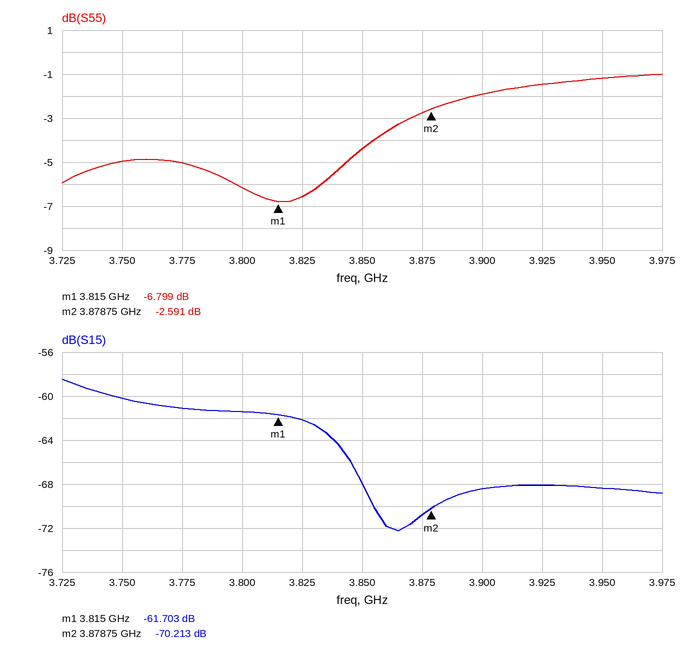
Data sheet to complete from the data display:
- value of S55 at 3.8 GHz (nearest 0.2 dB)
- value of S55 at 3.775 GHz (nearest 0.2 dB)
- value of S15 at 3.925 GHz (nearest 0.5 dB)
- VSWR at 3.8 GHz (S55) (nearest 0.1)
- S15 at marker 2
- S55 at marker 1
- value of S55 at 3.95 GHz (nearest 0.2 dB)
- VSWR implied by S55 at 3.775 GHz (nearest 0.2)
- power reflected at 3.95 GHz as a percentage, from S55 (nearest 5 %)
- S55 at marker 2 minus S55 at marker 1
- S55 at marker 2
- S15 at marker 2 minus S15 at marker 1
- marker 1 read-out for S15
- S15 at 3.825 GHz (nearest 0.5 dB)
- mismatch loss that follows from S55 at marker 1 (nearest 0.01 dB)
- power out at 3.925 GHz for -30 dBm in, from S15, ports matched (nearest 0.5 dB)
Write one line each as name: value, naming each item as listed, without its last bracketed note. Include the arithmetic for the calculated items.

value of S55 at 3.8 GHz: -6.2 dB
value of S55 at 3.775 GHz: -5.0 dB
value of S15 at 3.925 GHz: -68.0 dB
VSWR at 3.8 GHz (S55): |Γ| = 10^(-6.2/20) = 0.4898; VSWR = (1 + 0.4898)/(1 − 0.4898) ≈ 2.9
S15 at marker 2: -70.213 dB
S55 at marker 1: -6.799 dB
value of S55 at 3.95 GHz: -1.2 dB
VSWR implied by S55 at 3.775 GHz: |Γ| = 10^(-5/20) = 0.5623; VSWR = (1 + 0.5623)/(1 − 0.5623) ≈ 3.6
power reflected at 3.95 GHz as a percentage, from S55: 10^(-1.2/10) ≈ 75.9 %, so 75 % to the nearest 5 %
S55 at marker 2 minus S55 at marker 1: -2.591 − (-6.799) = 4.208 dB
S55 at marker 2: -2.591 dB
S15 at marker 2 minus S15 at marker 1: -70.213 − (-61.703) = -8.510 dB
marker 1 read-out for S15: -61.703 dB
S15 at 3.825 GHz: -62.0 dB
mismatch loss that follows from S55 at marker 1: −10 log10(1 − 10^(-6.799/10)) ≈ 1.02 dB
power out at 3.925 GHz for -30 dBm in, from S15, ports matched: -30 dBm + (-68.0 dB) = -98.0 dBm
